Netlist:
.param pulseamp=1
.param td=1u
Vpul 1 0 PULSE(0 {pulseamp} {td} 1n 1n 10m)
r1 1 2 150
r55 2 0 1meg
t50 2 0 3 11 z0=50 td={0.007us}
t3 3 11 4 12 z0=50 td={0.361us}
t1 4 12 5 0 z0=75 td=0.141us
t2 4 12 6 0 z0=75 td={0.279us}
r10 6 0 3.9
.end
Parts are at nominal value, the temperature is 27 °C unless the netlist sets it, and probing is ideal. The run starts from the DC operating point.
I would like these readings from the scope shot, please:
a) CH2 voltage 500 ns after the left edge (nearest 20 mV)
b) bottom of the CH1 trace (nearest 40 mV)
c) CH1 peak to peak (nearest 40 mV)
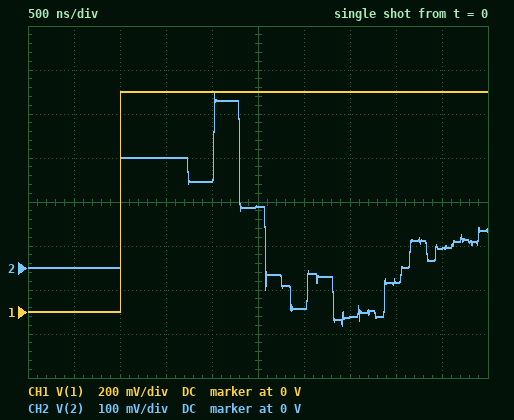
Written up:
0 V
0 V
1.00 V
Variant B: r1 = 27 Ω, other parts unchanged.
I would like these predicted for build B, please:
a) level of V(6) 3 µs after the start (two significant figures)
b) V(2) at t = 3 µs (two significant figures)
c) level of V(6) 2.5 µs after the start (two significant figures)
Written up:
96 mV
280 mV
98 mV
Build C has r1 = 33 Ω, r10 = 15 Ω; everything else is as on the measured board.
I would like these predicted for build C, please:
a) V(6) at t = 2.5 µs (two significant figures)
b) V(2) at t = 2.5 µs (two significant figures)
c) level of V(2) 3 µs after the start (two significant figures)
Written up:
290 mV
510 mV
350 mV
